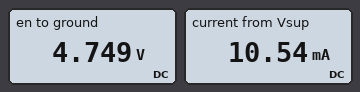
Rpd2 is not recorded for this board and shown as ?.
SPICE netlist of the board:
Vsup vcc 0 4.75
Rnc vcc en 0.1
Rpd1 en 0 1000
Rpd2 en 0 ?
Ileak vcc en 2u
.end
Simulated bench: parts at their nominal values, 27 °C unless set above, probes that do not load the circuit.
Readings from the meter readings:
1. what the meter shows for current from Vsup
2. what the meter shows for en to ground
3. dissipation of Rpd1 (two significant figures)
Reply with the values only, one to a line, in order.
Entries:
10.54 mA
4.749 V
23 mW
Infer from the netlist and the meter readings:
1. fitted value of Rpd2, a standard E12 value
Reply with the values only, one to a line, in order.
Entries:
820 Ω
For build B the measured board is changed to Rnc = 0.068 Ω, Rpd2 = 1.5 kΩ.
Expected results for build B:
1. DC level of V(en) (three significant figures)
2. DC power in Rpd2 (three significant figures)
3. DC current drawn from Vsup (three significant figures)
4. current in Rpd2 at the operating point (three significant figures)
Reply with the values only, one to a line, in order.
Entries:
4.75 V
15.0 mW
7.92 mA
3.17 mA
